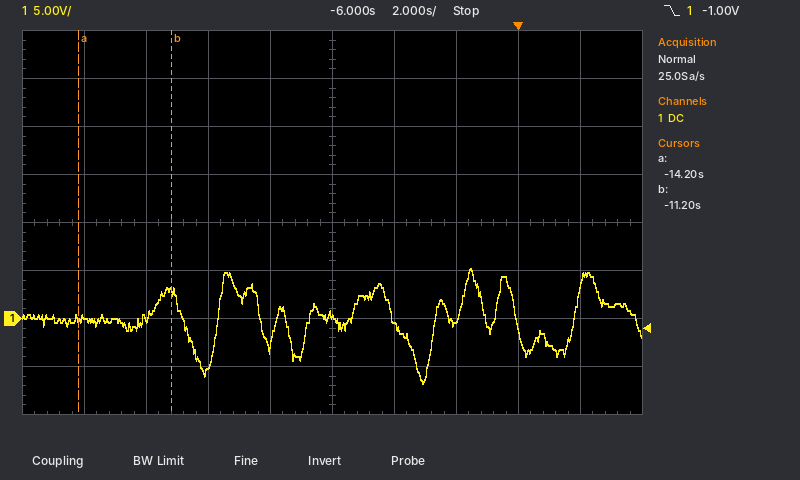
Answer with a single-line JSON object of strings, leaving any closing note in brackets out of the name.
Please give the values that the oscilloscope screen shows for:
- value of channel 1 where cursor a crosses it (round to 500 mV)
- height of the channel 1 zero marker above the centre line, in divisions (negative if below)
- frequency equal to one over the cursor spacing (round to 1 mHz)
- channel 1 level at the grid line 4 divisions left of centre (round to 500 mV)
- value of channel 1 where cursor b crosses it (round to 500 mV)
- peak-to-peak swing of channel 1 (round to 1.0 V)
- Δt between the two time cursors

{"value of channel 1 where cursor a crosses it": "0.0 V", "height of the channel 1 zero marker above the centre line, in divisions": "-2.0 div", "frequency equal to one over the cursor spacing": "333 mHz", "channel 1 level at the grid line 4 divisions left of centre": "0.0 V", "value of channel 1 where cursor b crosses it": "3.0 V", "peak-to-peak swing of channel 1": "12.0 V", "Δt between the two time cursors": "3.0 s"}
